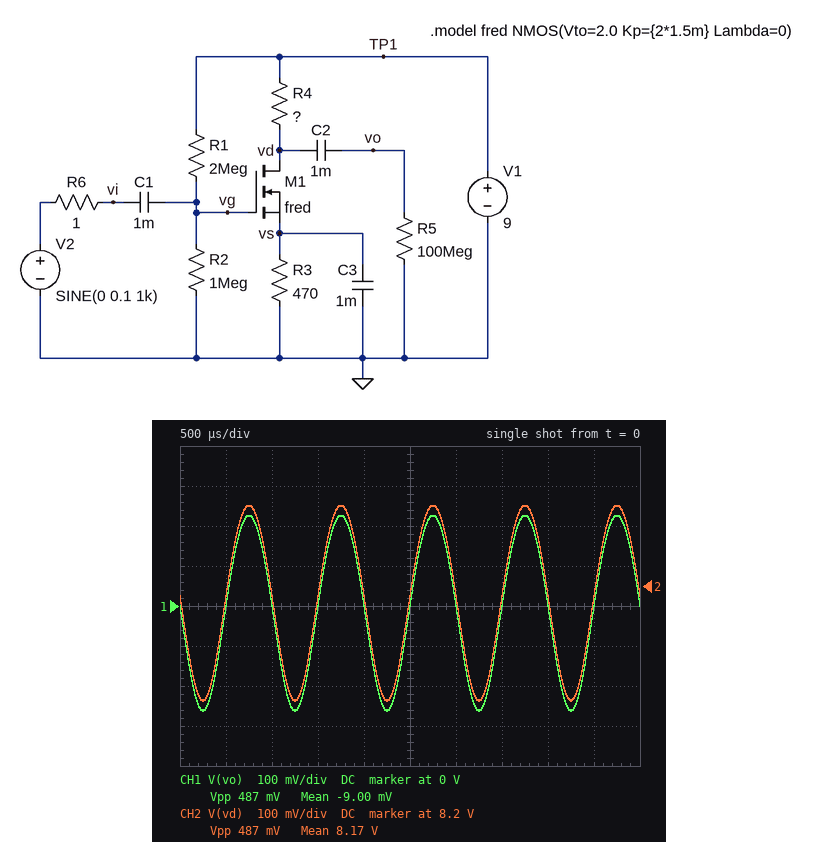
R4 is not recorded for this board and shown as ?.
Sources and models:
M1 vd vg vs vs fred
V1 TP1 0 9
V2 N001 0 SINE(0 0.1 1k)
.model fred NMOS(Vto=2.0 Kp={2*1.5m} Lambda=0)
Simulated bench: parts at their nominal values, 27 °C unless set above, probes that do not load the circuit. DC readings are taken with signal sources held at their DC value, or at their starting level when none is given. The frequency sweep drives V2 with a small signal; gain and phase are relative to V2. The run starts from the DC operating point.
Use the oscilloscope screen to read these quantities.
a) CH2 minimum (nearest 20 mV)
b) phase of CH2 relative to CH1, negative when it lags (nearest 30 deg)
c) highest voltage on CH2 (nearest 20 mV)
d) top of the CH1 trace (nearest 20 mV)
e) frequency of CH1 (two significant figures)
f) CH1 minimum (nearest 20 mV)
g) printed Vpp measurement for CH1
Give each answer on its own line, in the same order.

7.92 V
0 deg
8.40 V
220 mV
1.0 kHz
-260 mV
487 mV
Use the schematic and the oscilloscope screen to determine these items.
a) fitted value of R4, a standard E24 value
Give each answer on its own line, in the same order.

1.2 kΩ
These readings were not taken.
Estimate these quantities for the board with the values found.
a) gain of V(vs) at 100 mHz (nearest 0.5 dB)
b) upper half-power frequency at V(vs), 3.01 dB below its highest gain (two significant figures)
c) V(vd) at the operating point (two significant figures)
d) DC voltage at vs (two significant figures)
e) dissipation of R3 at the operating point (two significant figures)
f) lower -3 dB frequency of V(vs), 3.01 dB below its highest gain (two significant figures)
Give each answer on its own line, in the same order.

-6.5 dB
660 mHz
8.2 V
320 mV
220 µW
240 µHz
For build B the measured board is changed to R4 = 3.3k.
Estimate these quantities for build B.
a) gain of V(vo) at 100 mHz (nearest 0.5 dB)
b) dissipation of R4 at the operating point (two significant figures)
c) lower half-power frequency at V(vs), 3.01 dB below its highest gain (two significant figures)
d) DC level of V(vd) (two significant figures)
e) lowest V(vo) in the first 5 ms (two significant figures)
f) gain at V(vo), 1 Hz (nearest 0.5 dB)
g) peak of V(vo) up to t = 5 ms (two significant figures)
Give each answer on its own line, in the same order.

11.0 dB
1.6 mW
240 µHz
6.7 V
-720 mV
15.5 dB
620 mV
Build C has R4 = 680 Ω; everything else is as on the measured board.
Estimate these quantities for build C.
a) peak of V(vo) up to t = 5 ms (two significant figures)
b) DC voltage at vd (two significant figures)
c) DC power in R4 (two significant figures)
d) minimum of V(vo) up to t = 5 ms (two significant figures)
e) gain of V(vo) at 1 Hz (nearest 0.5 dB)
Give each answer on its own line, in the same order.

130 mV
8.5 V
320 µW
-150 mV
1.5 dB
